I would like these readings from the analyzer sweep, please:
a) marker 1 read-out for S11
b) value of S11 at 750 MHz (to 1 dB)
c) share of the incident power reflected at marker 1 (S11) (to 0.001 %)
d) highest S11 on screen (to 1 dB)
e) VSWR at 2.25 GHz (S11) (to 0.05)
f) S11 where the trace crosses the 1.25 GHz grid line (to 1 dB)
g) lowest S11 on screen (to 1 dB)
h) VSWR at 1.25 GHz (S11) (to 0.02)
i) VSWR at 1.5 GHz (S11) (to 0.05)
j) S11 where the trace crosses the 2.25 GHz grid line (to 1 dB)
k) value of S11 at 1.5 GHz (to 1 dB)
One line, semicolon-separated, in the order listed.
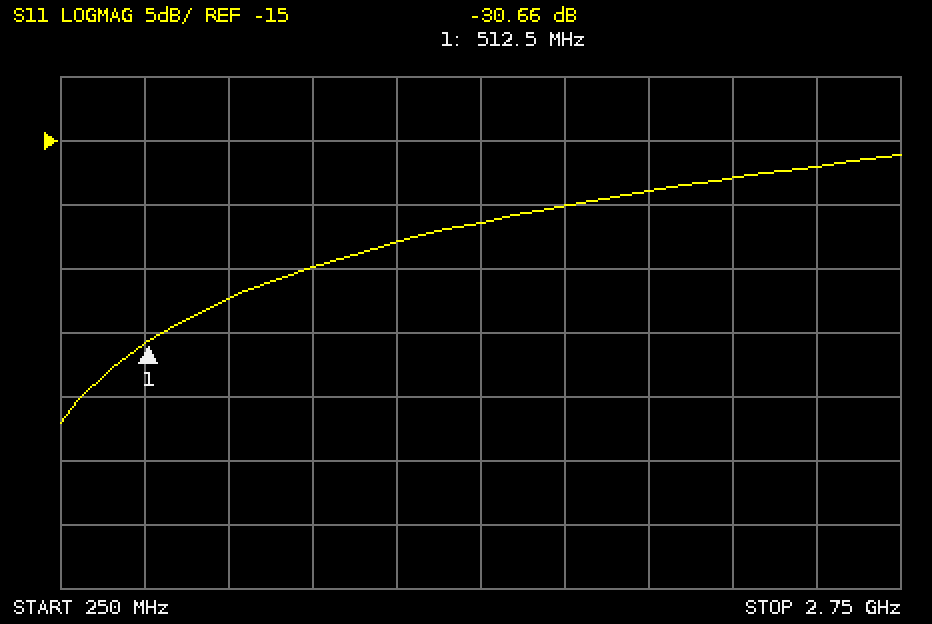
-30.66 dB; -27 dB; 0.086 %; -16 dB; 1.30; -23 dB; -37 dB; 1.16; 1.20; -18 dB; -21 dB
